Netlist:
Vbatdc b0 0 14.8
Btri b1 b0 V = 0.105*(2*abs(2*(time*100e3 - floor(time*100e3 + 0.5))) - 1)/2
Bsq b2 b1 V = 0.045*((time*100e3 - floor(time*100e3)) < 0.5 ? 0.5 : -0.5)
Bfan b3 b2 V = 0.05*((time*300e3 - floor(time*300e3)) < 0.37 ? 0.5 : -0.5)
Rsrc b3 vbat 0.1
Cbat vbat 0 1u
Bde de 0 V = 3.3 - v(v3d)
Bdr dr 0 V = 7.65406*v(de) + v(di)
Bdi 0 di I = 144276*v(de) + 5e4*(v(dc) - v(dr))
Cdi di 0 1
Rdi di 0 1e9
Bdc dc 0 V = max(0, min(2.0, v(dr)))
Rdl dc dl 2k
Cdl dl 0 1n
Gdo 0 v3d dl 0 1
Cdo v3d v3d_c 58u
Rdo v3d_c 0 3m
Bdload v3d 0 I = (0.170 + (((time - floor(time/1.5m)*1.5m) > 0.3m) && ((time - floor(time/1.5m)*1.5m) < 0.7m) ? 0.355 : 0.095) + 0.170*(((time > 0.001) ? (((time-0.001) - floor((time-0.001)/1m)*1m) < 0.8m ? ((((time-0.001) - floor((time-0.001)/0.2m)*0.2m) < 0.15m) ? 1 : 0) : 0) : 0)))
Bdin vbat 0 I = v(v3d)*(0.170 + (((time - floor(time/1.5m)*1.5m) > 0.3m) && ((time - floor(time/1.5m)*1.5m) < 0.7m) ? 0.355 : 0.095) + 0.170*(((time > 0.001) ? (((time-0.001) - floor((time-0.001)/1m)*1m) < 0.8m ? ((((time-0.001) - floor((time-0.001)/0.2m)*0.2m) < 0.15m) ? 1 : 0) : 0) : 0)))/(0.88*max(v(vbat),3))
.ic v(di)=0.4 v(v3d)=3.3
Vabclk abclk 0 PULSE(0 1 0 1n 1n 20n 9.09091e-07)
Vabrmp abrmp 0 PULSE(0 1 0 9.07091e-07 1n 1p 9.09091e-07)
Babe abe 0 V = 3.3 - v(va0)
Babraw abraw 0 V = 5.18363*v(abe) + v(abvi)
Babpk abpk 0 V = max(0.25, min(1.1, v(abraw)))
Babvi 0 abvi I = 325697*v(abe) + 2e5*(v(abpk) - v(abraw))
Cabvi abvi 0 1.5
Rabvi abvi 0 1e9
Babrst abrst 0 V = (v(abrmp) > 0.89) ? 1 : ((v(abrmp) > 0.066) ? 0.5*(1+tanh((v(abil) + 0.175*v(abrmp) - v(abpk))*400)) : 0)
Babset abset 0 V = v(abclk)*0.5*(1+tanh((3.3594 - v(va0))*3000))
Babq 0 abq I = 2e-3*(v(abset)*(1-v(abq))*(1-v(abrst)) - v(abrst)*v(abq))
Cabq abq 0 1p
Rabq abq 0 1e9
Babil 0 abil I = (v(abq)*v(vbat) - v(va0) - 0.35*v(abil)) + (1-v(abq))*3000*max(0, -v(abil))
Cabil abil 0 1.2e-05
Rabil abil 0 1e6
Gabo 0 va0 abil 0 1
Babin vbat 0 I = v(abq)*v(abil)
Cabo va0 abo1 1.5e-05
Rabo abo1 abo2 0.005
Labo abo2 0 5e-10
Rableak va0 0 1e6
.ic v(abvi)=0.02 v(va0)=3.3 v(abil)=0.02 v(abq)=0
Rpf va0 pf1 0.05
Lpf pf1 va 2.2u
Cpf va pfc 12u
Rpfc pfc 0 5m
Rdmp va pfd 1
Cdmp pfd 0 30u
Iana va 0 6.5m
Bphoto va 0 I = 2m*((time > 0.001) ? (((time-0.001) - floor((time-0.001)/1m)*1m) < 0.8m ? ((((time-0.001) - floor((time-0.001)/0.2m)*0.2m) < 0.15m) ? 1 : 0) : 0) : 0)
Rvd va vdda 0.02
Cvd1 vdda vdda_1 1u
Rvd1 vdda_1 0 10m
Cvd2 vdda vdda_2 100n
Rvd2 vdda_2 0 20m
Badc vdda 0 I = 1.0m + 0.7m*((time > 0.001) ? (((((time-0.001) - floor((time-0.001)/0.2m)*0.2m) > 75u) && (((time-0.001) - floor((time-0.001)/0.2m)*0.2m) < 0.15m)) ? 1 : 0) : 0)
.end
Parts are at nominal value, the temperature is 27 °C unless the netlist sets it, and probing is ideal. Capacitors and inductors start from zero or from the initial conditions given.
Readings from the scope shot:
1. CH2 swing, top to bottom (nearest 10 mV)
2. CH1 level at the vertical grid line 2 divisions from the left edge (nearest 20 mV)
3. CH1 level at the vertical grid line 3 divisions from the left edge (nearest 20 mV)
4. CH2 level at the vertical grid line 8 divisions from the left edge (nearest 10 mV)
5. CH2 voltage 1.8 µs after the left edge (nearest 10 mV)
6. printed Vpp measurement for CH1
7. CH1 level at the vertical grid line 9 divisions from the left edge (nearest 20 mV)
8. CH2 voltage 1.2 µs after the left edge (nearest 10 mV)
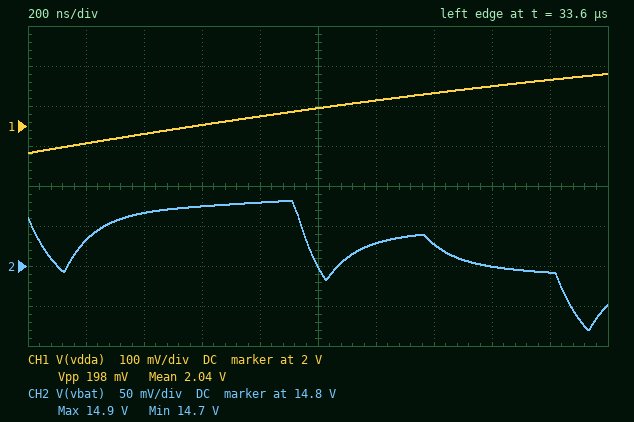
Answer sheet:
160 mV
1.98 V
2.00 V
14.80 V
14.79 V
198 mV
2.12 V
14.83 V
